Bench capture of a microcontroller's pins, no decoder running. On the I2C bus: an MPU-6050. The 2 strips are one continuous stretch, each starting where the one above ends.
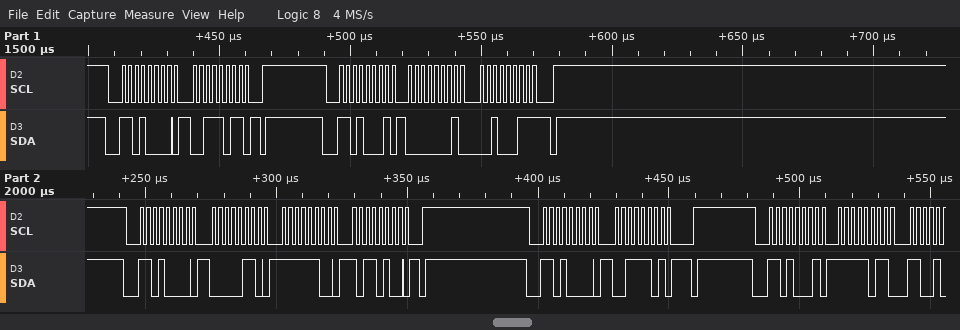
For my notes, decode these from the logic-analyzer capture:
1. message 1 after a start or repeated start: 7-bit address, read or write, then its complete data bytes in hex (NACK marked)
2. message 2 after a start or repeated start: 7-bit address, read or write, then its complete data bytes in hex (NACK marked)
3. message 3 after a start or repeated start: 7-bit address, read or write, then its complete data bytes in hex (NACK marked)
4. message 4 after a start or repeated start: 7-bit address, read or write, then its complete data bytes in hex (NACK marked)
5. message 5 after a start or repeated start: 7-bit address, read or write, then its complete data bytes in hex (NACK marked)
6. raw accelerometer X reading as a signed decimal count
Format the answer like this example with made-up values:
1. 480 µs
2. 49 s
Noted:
1. 0x68 write: 3B
2. 0x68 read: 01 23 NACK
3. 0x68 write: 06 FC B4
4. 0x68 write: 3D
5. 0x68 read: FB
6. 291
